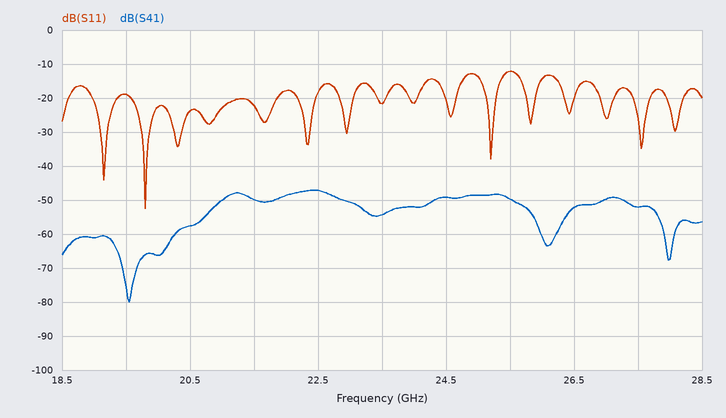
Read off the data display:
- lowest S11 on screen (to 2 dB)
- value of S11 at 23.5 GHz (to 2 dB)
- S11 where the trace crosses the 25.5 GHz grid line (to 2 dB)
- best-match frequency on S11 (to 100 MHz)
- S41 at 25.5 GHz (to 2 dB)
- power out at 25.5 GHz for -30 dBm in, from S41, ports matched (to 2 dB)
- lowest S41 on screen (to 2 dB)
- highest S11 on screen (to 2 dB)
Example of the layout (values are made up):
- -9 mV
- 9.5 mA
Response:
- -52 dB
- -22 dB
- -12 dB
- 19.8 GHz
- -50 dB
- -80 dBm
- -80 dB
- -12 dB
